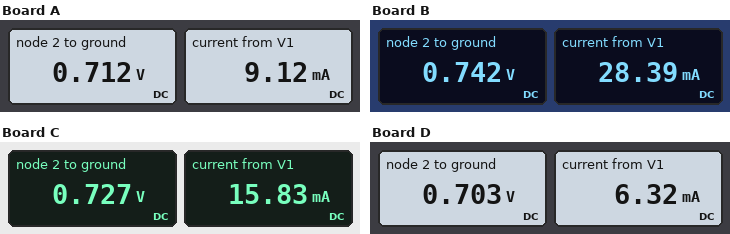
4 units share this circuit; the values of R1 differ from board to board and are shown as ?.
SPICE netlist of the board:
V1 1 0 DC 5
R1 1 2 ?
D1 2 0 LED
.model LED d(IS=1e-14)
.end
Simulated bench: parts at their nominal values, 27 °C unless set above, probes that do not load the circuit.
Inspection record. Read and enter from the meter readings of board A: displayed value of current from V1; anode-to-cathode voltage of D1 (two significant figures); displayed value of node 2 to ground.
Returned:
9.12 mA
710 mV
0.712 V
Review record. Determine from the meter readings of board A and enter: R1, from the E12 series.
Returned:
470 Ω
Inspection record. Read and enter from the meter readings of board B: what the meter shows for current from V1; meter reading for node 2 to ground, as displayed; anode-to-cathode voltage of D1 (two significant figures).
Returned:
28.39 mA
0.742 V
740 mV
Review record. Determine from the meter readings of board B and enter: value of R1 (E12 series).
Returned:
150 Ω
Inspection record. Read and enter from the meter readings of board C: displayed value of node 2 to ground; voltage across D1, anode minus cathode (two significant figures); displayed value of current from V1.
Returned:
0.727 V
730 mV
15.83 mA
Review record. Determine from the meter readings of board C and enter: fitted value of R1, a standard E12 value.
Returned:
270 Ω
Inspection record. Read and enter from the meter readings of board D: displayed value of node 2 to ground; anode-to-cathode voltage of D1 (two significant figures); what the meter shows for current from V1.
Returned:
0.703 V
700 mV
6.32 mA
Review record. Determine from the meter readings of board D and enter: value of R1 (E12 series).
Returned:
680 Ω
